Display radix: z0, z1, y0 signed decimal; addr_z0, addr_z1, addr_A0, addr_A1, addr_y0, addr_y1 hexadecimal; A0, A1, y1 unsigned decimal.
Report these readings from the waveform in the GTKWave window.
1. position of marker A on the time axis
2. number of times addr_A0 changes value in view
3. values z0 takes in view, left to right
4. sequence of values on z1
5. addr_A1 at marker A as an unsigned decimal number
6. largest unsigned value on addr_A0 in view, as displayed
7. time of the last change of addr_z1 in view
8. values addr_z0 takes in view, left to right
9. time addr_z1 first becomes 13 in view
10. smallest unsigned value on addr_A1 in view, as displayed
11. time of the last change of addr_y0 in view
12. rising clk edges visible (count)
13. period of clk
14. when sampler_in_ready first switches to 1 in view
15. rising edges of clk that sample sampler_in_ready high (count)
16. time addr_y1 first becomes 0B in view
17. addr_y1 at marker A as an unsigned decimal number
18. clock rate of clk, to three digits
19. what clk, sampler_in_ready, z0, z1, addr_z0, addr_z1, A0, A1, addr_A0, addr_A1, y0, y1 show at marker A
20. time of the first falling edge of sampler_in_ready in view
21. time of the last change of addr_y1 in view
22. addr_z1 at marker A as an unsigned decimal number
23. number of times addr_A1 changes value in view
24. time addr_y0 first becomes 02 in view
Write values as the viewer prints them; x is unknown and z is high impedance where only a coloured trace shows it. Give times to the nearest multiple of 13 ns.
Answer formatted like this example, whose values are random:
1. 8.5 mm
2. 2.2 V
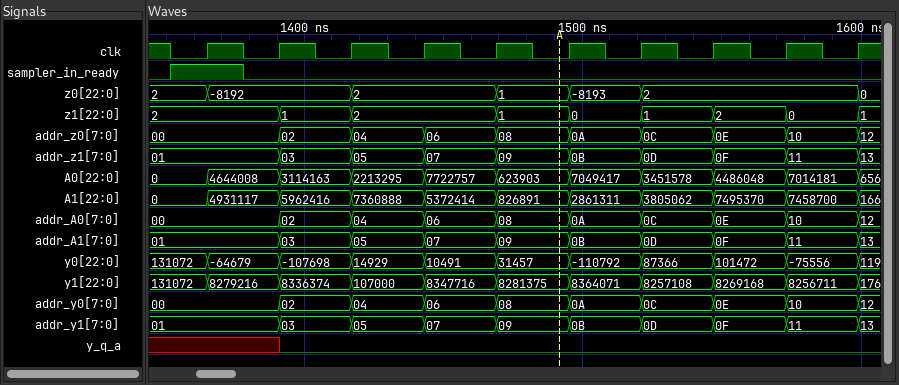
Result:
1. 1495 ns
2. 9
3. 2, -8192, 2, 1, -8193, 2, 0
4. 2, 1, 2, 1, 0, 1, 2, 0, 1
5. 9
6. 12
7. 1599 ns
8. 00, 02, 04, 06, 08, 0A, 0C, 0E, 10, 12
9. 1599 ns
10. 01
11. 1599 ns
12. 10
13. 26 ns
14. 1352 ns
15. 1
16. 1495 ns
17. 9
18. 38.5 MHz
19. clk=0, sampler_in_ready=0, z0=1, z1=1, addr_z0=08, addr_z1=09, A0=623903, A1=826891, addr_A0=08, addr_A1=09, y0=31457, y1=8281375
20. 1378 ns
21. 1599 ns
22. 9
23. 9
24. 1391 ns
